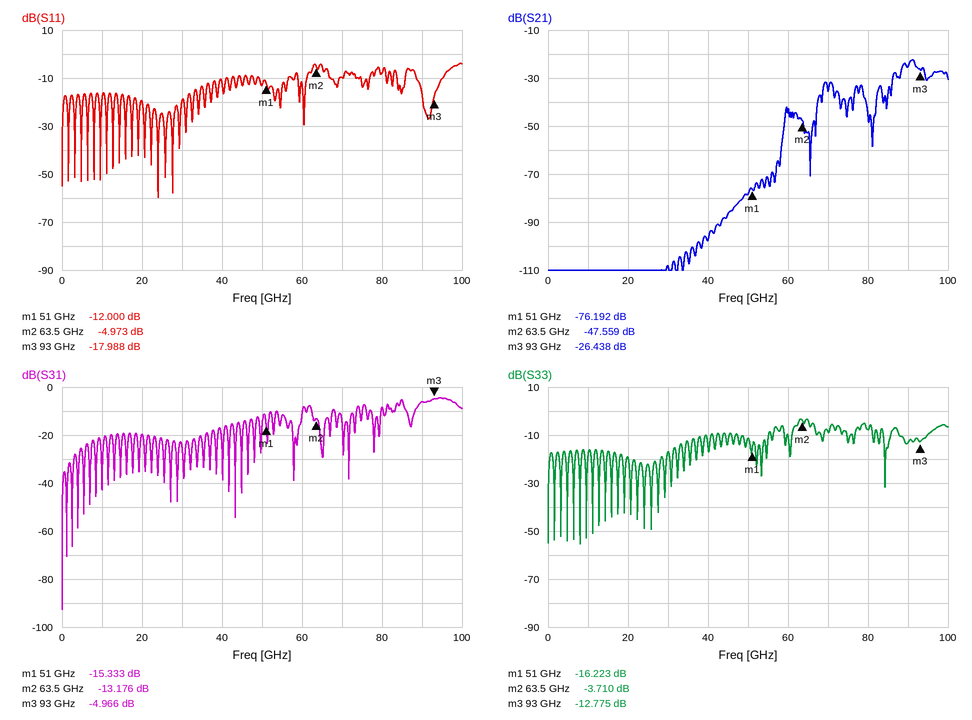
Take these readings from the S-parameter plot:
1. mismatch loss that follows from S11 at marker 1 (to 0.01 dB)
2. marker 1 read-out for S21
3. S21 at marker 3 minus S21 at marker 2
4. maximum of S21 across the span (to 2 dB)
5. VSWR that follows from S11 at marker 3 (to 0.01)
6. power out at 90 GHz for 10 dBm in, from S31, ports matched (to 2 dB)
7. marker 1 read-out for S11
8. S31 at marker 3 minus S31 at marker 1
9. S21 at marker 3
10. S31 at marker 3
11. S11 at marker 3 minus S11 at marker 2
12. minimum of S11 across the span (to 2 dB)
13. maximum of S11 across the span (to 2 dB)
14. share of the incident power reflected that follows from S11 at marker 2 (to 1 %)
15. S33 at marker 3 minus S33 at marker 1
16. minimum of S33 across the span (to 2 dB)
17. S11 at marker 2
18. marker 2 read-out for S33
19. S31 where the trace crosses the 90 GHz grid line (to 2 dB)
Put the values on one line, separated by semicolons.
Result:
0.28 dB; -76.192 dB; 21.121 dB; -22 dB; 1.29; 4 dBm; -12.000 dB; 10.367 dB; -26.438 dB; -4.966 dB; -13.015 dB; -60 dB; -4 dB; 32 %; 3.448 dB; -56 dB; -4.973 dB; -3.710 dB; -6 dB
